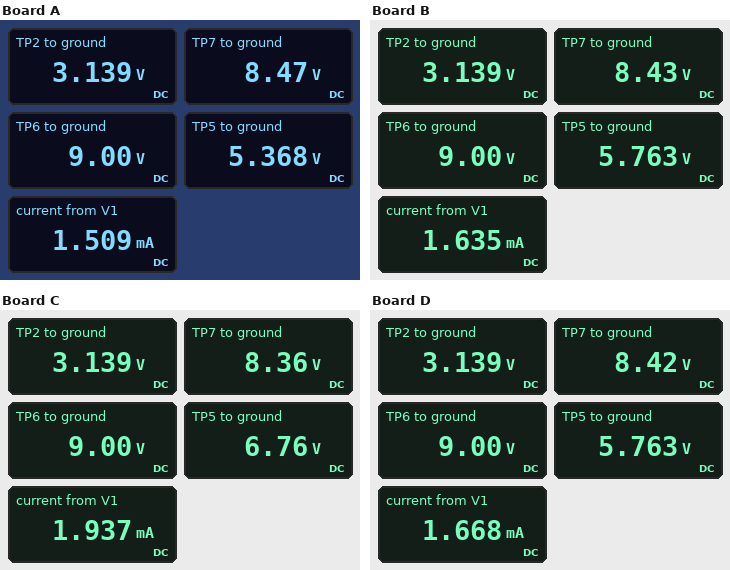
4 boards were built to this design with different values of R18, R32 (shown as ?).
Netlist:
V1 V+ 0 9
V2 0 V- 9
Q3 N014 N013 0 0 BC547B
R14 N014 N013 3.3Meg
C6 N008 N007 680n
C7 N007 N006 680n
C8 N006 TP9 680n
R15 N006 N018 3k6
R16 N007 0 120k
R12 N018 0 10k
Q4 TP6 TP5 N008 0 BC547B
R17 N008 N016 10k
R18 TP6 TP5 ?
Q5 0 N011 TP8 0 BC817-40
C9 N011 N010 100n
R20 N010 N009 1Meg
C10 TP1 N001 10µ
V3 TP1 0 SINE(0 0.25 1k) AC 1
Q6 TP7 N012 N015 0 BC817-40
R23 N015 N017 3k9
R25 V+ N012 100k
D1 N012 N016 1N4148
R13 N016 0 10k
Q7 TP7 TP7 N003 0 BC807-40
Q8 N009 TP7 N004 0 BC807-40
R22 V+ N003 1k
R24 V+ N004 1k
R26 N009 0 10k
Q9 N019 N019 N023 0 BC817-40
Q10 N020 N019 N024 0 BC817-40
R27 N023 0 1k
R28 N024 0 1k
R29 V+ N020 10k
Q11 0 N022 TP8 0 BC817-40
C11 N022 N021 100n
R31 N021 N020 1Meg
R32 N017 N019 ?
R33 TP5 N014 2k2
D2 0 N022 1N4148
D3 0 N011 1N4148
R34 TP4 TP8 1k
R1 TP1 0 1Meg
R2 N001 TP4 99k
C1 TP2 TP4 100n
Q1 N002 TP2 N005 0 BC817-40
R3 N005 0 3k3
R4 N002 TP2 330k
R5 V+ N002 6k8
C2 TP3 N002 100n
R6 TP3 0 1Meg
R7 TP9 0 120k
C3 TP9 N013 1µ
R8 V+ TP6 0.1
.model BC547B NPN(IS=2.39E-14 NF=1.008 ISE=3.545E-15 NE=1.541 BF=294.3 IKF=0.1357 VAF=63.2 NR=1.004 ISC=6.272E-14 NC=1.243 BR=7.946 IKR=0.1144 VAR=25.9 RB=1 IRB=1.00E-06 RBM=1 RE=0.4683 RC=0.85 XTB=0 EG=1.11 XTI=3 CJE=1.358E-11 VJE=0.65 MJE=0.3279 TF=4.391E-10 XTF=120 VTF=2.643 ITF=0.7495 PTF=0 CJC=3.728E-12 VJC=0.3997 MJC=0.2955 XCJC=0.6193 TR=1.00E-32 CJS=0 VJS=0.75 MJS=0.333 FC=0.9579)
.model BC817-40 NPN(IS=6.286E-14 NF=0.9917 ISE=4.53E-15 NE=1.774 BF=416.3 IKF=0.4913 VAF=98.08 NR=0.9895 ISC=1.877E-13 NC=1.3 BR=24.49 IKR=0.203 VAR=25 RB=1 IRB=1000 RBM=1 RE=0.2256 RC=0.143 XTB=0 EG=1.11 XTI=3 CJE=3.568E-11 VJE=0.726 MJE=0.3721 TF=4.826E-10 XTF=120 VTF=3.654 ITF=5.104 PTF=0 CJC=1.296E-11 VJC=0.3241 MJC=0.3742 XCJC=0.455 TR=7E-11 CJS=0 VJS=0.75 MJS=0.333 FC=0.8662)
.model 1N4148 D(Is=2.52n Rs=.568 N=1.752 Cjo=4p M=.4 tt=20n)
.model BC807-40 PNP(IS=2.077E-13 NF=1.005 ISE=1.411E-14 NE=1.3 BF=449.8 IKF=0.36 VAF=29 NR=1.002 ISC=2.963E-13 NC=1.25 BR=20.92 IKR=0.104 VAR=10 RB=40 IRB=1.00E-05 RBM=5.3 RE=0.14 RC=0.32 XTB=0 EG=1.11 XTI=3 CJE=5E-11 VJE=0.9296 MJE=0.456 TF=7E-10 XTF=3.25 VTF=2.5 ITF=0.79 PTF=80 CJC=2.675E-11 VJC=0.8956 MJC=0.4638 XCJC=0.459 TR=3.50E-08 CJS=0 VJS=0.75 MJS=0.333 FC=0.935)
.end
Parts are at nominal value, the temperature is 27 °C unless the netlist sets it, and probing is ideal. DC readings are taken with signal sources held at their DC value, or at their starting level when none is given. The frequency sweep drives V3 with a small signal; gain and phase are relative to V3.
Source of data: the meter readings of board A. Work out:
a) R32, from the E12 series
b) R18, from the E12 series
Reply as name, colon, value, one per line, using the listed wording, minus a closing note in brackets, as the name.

R32, from the E12 series: 56 kΩ
R18, from the E12 series: 10 kΩ
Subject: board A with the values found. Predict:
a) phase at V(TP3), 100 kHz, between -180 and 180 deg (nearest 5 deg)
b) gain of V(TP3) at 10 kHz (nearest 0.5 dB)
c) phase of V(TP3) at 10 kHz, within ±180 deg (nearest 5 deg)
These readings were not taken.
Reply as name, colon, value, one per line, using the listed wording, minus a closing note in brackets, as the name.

phase at V(TP3), 100 kHz, between -180 and 180 deg: 120 deg
gain of V(TP3) at 10 kHz: -0.5 dB
phase of V(TP3) at 10 kHz, within ±180 deg: 170 deg
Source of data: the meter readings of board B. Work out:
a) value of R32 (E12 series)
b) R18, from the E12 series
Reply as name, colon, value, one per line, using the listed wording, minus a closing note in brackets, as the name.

value of R32: 33 kΩ
R18, from the E12 series: 8.2 kΩ
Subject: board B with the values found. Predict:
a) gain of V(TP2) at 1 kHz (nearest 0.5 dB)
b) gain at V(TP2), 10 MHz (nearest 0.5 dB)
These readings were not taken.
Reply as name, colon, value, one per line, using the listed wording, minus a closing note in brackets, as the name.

gain of V(TP2) at 1 kHz: -6.0 dB
gain at V(TP2), 10 MHz: -42.0 dB
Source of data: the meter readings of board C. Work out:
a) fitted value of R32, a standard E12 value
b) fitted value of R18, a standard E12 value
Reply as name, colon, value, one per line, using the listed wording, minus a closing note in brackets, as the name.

fitted value of R32, a standard E12 value: 18 kΩ
fitted value of R18, a standard E12 value: 4.7 kΩ
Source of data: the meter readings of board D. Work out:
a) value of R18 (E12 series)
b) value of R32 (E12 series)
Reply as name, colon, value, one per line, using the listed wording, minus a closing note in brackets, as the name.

value of R18: 8.2 kΩ
value of R32: 27 kΩ
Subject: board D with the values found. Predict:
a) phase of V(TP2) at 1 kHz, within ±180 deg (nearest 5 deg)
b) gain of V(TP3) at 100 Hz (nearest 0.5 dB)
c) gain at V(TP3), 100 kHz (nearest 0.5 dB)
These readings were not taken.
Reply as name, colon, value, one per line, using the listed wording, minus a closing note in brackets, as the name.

phase of V(TP2) at 1 kHz, within ±180 deg: 0 deg
gain of V(TP3) at 100 Hz: 0 dB
gain at V(TP3), 100 kHz: -5.5 dB
